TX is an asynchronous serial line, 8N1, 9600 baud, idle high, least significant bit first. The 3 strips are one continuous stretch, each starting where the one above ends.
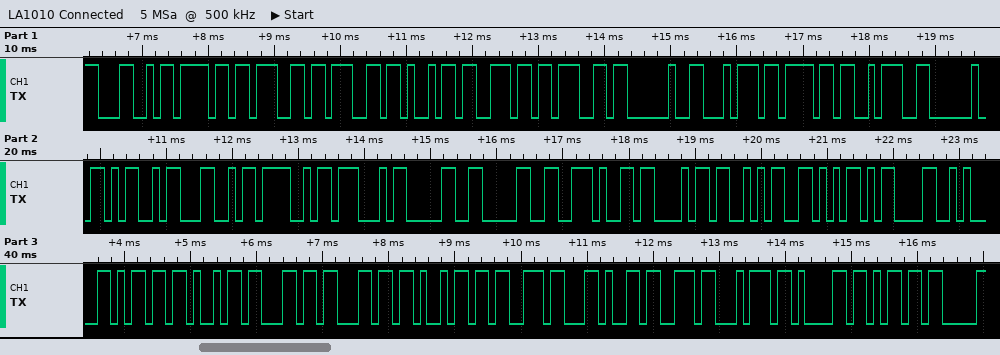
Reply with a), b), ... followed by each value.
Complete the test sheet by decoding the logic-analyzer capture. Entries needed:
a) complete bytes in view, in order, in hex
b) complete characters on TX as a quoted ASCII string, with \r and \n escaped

a) 4C 6F 67 67 69 6E 67 20 74 6F 3A 20 4D 4C 4F 47 30 30 2E 43 53 56 0D 0A 6D 69 6C 6C 69 73 2C 73 74 61 6D
b) "Logging to: MLOG00.CSV\r\nmillis,stam"
